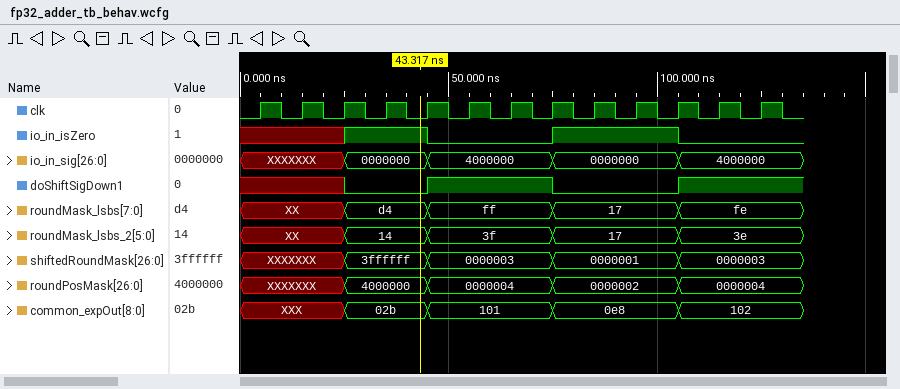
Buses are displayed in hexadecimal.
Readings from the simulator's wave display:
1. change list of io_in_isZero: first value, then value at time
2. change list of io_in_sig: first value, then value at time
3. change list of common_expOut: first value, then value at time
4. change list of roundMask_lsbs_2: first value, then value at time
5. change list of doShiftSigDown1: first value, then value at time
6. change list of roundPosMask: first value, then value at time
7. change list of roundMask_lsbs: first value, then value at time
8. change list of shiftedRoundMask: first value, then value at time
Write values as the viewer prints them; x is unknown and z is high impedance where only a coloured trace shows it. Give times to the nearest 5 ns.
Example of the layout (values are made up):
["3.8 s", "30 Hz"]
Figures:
["x, 1 at 25 ns, 0 at 45 ns, 1 at 75 ns, 0 at 105 ns", "XXXXXXX, 0000000 at 25 ns, 4000000 at 45 ns, 0000000 at 75 ns, 4000000 at 105 ns", "XXX, 02b at 25 ns, 101 at 45 ns, 0e8 at 75 ns, 102 at 105 ns", "XX, 14 at 25 ns, 3f at 45 ns, 17 at 75 ns, 3e at 105 ns", "x, 0 at 25 ns, 1 at 45 ns, 0 at 75 ns, 1 at 105 ns", "XXXXXXX, 4000000 at 25 ns, 0000004 at 45 ns, 0000002 at 75 ns, 0000004 at 105 ns", "XX, d4 at 25 ns, ff at 45 ns, 17 at 75 ns, fe at 105 ns", "XXXXXXX, 3ffffff at 25 ns, 0000003 at 45 ns, 0000001 at 75 ns, 0000003 at 105 ns"]
